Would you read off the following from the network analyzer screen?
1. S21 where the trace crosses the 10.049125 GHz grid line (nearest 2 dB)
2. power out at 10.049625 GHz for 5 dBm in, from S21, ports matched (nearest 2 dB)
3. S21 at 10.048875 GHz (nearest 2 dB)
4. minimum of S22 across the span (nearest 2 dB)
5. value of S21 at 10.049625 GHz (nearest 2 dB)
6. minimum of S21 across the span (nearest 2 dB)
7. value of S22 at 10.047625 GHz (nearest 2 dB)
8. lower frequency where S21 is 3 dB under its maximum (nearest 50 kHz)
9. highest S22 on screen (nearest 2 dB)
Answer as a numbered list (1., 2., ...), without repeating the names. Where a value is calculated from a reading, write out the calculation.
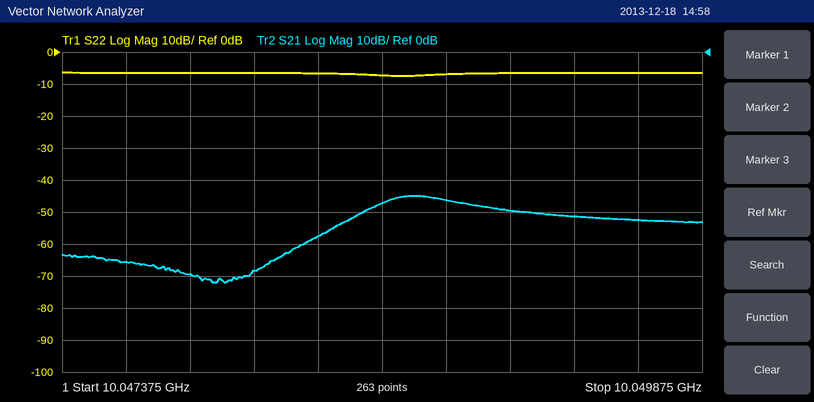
1. -50 dB
2. 5 dBm + (-52 dB) = -48 dBm
3. -46 dB
4. -8 dB
5. -52 dB
6. -72 dB
7. -6 dB
8. 10.04860 GHz
9. -6 dB
